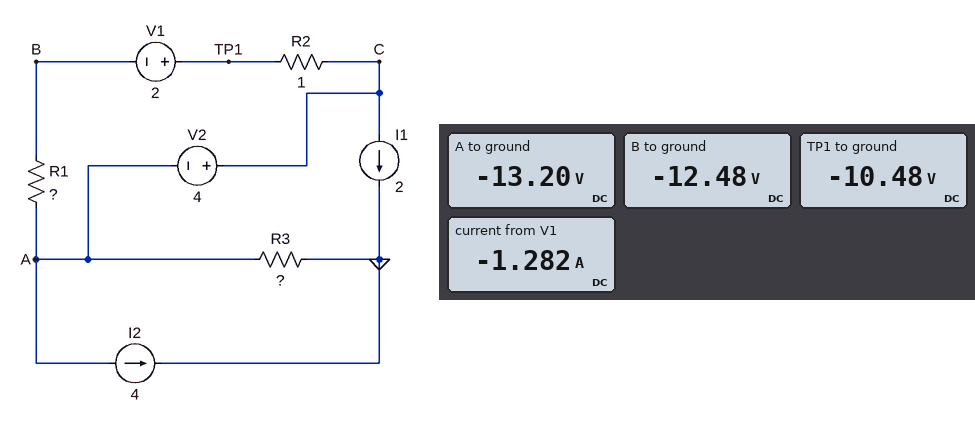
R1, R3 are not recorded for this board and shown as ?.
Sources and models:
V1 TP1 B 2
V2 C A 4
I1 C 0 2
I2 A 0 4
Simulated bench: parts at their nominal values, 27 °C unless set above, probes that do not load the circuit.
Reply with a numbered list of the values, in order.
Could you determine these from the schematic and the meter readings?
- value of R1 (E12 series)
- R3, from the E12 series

1. 0.56 Ω
2. 2.2 Ω
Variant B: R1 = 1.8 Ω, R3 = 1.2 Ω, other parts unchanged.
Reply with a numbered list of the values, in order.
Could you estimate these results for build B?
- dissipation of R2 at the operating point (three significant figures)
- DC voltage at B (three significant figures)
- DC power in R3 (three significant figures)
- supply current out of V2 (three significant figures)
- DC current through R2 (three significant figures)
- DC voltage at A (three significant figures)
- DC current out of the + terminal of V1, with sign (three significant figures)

1. 510 mW
2. -5.91 V
3. 43.2 W
4. 2.71 A
5. 714 mA
6. -7.20 V
7. -714 mA
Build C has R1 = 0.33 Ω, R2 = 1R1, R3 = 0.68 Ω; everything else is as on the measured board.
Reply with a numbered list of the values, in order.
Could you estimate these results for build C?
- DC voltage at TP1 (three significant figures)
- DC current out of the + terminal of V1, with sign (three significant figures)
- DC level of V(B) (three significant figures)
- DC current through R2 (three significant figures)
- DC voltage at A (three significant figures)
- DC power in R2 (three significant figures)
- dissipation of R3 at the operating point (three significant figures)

1. -1.62 V
2. -1.40 A
3. -3.62 V
4. 1.40 A
5. -4.08 V
6. 2.15 W
7. 24.5 W
